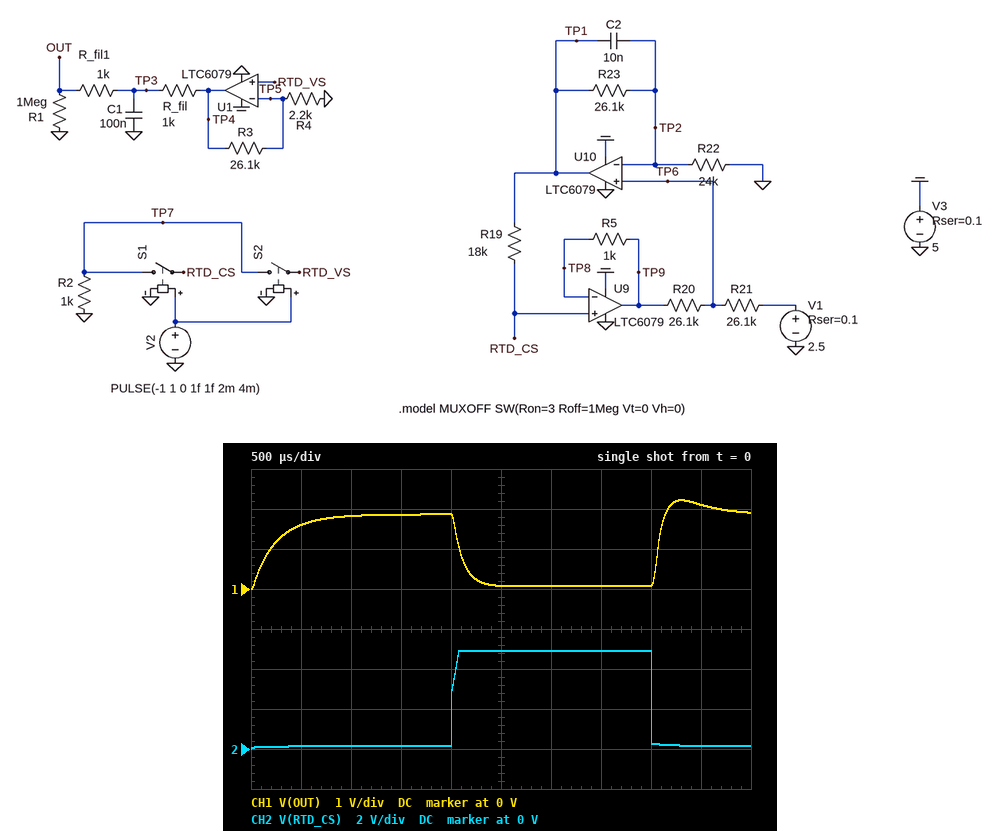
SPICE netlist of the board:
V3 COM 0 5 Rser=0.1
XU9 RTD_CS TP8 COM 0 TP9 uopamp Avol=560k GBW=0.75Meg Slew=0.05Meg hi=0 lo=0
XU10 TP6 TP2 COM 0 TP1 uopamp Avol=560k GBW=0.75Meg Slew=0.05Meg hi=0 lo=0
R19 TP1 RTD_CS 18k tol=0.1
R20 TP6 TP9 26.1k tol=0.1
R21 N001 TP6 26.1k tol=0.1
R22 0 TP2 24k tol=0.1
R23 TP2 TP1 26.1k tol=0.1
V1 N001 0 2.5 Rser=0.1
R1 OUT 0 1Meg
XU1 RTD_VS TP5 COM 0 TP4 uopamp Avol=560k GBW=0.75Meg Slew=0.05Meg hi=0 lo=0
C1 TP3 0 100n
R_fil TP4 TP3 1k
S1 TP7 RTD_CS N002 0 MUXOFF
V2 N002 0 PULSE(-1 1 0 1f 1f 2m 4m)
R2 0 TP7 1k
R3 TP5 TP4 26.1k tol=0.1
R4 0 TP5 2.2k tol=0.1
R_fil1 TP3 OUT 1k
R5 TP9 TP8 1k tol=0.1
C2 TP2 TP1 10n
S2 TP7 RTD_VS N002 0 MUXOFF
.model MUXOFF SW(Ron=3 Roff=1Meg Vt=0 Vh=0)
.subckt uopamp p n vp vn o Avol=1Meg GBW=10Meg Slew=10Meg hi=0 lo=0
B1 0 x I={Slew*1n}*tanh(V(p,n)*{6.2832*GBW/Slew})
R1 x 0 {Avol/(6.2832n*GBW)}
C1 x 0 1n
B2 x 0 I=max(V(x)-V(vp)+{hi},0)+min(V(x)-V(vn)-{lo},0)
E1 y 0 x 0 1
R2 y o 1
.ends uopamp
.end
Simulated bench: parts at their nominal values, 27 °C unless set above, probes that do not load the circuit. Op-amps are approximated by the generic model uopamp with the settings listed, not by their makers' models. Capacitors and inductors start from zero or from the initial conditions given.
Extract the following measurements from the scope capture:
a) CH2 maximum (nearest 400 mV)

4.8 V
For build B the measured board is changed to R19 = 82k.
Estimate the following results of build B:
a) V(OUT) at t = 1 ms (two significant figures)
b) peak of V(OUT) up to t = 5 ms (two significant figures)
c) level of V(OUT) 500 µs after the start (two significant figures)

400 mV
510 mV
350 mV
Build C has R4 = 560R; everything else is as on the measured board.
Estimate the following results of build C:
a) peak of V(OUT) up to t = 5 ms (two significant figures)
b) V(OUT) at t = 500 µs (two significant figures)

5.0 V
4.9 V
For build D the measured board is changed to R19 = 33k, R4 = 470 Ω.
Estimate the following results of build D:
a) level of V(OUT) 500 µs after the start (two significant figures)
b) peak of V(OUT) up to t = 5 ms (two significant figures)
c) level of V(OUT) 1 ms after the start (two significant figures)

3.8 V
4.9 V
4.4 V
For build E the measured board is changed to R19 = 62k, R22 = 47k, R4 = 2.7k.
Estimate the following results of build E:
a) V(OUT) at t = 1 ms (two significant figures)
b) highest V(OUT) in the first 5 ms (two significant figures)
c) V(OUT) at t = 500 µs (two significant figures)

330 mV
440 mV
300 mV
